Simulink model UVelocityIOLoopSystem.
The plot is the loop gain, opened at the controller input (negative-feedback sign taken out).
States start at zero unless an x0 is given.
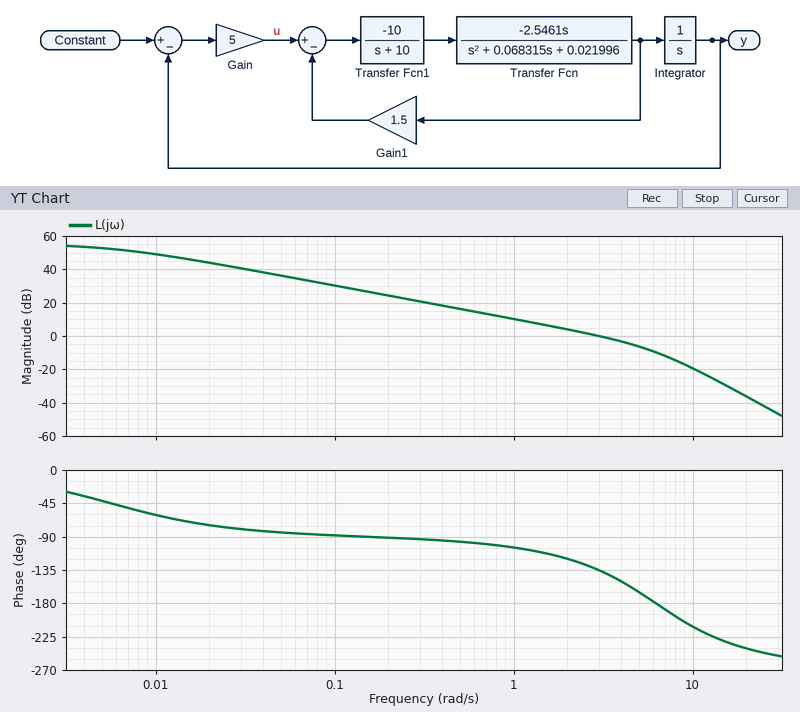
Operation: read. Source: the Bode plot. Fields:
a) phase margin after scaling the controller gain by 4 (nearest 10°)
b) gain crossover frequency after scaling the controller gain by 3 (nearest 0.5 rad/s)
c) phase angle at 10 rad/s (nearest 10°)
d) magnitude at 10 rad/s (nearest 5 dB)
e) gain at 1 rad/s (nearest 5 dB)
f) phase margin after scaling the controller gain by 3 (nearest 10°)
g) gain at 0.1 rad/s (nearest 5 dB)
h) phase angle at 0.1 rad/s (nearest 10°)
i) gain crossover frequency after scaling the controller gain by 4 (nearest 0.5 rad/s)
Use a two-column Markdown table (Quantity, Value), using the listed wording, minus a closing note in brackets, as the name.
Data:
| Quantity | Value |
|---|---|
| phase margin after scaling the controller gain by 4 | -10° |
| gain crossover frequency after scaling the controller gain by 3 | 6.0 rad/s |
| phase angle at 10 rad/s | -210° |
| magnitude at 10 rad/s | -20 dB |
| gain at 1 rad/s | 10 dB |
| phase margin after scaling the controller gain by 3 | 0° |
| gain at 0.1 rad/s | 30 dB |
| phase angle at 0.1 rad/s | -90° |
| gain crossover frequency after scaling the controller gain by 4 | 7.0 rad/s |
